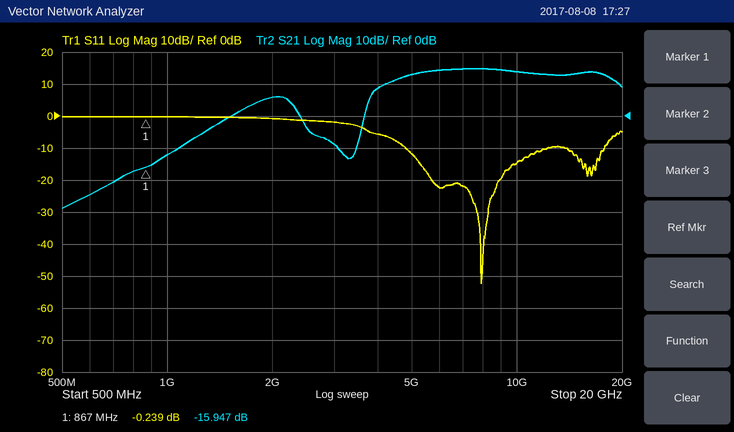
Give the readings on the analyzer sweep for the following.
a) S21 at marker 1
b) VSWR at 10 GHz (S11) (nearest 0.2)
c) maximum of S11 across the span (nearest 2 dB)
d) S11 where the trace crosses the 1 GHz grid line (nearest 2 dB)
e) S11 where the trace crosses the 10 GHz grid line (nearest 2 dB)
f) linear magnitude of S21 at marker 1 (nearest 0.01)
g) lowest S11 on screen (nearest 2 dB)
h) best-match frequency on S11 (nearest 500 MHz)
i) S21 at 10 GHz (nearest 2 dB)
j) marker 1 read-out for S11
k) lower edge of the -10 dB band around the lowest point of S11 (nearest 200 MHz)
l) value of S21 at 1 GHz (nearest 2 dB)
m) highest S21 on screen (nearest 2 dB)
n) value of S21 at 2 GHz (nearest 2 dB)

-15.947 dB
1.4
0 dB
0 dB
-14 dB
0.16
-52 dB
8.0 GHz
14 dB
-0.239 dB
4.8 GHz
-12 dB
14 dB
6 dB
